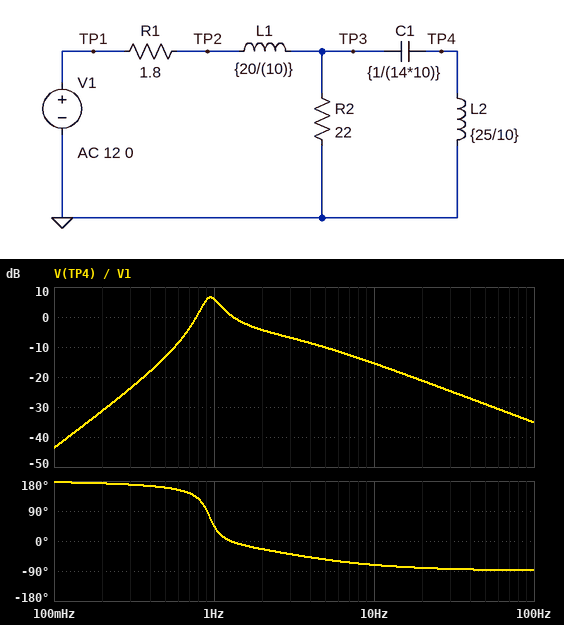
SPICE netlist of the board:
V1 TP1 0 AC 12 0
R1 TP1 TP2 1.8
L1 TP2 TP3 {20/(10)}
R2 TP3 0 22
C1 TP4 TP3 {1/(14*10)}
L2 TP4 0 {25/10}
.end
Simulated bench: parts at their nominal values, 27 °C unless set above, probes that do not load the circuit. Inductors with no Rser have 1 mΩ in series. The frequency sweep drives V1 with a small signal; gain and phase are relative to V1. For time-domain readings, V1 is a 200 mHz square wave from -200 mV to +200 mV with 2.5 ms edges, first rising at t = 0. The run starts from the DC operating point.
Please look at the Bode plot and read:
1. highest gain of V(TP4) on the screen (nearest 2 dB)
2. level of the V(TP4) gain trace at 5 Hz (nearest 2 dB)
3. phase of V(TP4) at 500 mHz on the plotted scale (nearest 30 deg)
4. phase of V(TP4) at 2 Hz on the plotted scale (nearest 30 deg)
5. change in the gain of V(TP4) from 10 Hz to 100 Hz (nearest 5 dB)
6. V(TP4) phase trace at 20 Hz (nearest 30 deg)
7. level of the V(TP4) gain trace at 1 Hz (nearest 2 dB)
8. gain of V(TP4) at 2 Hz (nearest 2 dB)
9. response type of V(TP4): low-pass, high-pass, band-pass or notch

6 dB
-10 dB
150 deg
-30 deg
-20 dB
-90 deg
6 dB
-4 dB
band-pass
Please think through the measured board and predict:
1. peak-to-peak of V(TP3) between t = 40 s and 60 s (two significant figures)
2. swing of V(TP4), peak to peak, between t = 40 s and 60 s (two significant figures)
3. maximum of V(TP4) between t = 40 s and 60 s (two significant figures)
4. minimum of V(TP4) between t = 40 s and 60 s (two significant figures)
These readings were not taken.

570 mV
370 mV
190 mV
-190 mV
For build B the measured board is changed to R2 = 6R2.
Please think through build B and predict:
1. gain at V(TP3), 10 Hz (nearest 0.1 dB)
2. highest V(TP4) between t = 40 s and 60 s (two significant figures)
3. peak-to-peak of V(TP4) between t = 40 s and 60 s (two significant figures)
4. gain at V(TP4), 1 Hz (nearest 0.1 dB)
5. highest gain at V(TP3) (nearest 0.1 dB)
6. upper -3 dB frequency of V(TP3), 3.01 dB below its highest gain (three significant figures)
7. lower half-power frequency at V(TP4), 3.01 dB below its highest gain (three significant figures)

-26.2 dB
99 mV
200 mV
0 dB
-2.2 dB
779 mHz
986 mHz
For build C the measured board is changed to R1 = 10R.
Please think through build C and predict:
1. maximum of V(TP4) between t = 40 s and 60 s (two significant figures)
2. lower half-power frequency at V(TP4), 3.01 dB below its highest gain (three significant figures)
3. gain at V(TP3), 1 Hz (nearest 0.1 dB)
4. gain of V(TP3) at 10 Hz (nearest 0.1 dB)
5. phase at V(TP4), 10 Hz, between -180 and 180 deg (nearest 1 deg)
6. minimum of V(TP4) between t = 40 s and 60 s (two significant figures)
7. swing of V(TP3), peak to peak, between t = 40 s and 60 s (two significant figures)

140 mV
877 mHz
-6.6 dB
-15.7 dB
-68 deg
-140 mV
380 mV
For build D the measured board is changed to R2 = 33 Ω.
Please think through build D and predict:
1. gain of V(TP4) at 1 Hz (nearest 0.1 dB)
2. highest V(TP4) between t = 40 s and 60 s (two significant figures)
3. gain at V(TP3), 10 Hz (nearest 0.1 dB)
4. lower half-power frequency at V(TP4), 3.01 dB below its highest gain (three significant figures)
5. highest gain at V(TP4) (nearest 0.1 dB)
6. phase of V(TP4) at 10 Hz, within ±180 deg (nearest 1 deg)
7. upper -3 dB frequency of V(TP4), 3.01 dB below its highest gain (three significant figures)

6.9 dB
200 mV
-12.5 dB
842 mHz
8.6 dB
-64 deg
1.04 Hz
